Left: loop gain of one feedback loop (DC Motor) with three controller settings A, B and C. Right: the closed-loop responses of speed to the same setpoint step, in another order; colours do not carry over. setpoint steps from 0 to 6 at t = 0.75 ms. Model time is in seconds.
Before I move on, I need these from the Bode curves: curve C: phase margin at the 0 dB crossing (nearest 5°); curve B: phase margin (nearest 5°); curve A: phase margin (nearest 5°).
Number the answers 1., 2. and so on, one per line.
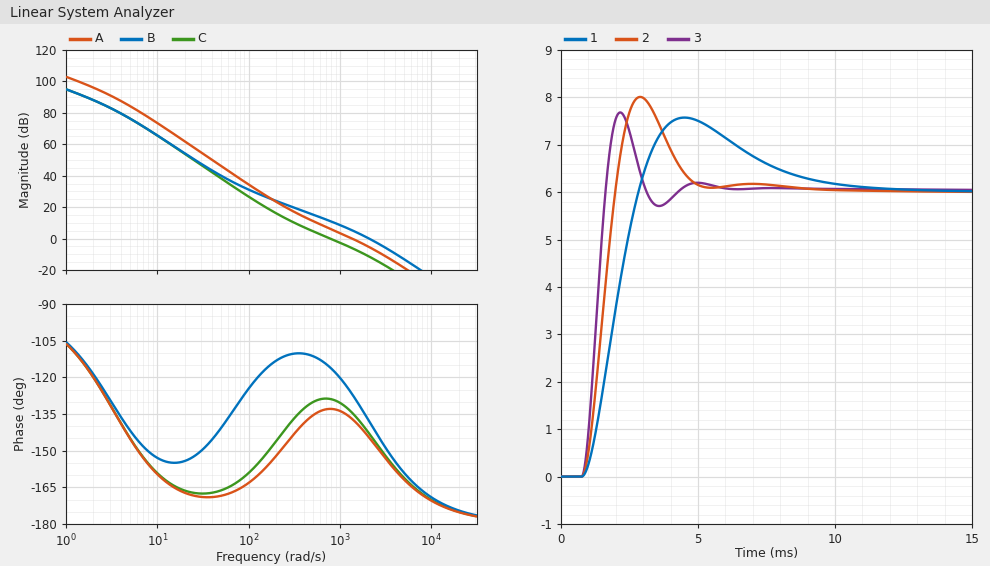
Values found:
1. 50°
2. 40°
3. 45°
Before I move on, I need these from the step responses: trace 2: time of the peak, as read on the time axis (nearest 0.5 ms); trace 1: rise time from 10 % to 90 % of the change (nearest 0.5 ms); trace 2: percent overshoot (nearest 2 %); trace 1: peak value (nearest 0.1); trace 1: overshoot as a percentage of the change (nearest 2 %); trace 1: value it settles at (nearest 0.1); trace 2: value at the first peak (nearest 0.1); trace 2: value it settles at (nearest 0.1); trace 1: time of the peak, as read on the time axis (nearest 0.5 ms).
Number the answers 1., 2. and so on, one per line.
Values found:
1. 3.0 ms
2. 1.5 ms
3. 34 %
4. 7.6
5. 26 %
6. 6.0
7. 8.0
8. 6.0
9. 4.5 ms
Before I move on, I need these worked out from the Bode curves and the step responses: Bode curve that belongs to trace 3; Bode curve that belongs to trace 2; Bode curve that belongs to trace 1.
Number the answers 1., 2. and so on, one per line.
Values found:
1. B
2. A
3. C
